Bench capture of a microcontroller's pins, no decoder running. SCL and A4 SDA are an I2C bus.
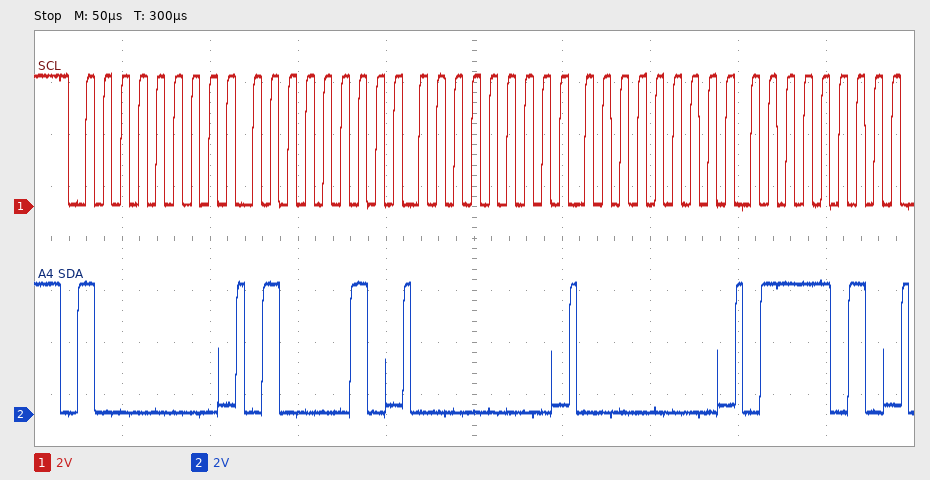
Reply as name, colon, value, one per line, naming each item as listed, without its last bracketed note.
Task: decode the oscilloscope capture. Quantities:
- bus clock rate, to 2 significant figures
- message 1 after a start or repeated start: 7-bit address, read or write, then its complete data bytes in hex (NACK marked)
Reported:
bus clock rate, to 2 significant figures: 100 kHz
message 1 after a start or repeated start: 7-bit address, read or write, then its complete data bytes in hex: 0x40 write: 42 00 00 7A
